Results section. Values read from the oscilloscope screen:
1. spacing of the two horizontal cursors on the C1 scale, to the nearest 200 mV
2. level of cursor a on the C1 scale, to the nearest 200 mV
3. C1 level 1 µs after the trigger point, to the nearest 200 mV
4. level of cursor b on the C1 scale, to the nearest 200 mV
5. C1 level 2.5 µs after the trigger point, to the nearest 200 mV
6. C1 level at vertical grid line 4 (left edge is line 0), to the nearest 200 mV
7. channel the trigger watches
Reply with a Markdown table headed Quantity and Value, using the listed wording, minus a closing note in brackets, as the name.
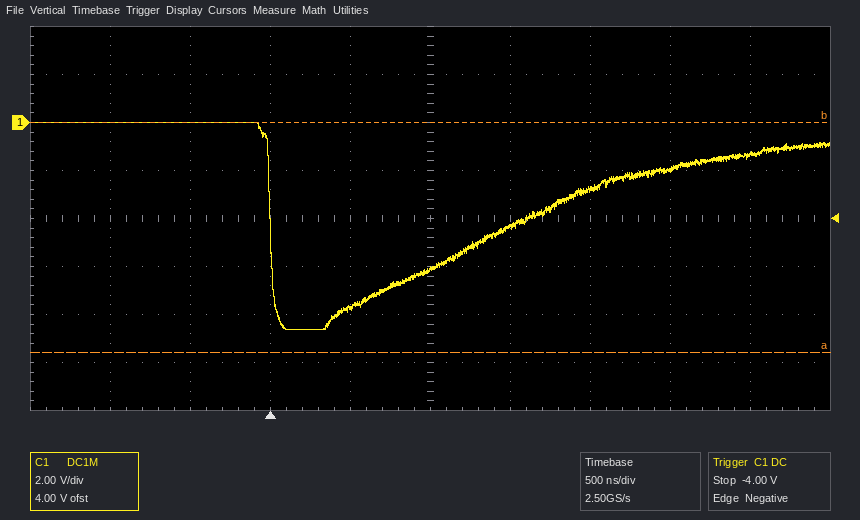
| Quantity | Value |
|---|---|
| spacing of the two horizontal cursors on the C1 scale, to the nearest 200 mV | 9.6 V |
| level of cursor a on the C1 scale, to the nearest 200 mV | -9.6 V |
| C1 level 1 µs after the trigger point, to the nearest 200 mV | -6.2 V |
| level of cursor b on the C1 scale, to the nearest 200 mV | 0.0 V |
| C1 level 2.5 µs after the trigger point, to the nearest 200 mV | -2.0 V |
| C1 level at vertical grid line 4 (left edge is line 0), to the nearest 200 mV | -7.8 V |
| channel the trigger watches | C1 |
